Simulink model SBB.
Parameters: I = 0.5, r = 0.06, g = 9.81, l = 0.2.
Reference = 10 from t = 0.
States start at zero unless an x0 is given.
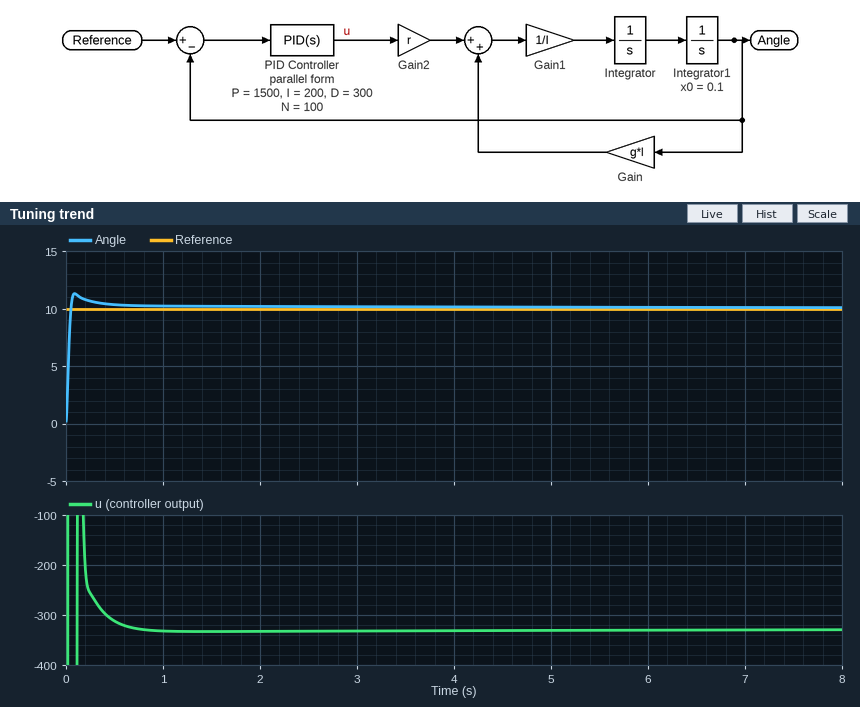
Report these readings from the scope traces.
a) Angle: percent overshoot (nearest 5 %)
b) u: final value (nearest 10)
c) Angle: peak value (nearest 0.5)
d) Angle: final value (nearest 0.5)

15 %
-330
11.5
10.0
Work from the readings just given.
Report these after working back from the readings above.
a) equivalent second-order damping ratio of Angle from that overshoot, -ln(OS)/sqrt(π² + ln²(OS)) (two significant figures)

0.52
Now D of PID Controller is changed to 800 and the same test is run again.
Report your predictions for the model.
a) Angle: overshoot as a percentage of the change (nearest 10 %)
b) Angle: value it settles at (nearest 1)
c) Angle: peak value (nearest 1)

20 %
10
12
